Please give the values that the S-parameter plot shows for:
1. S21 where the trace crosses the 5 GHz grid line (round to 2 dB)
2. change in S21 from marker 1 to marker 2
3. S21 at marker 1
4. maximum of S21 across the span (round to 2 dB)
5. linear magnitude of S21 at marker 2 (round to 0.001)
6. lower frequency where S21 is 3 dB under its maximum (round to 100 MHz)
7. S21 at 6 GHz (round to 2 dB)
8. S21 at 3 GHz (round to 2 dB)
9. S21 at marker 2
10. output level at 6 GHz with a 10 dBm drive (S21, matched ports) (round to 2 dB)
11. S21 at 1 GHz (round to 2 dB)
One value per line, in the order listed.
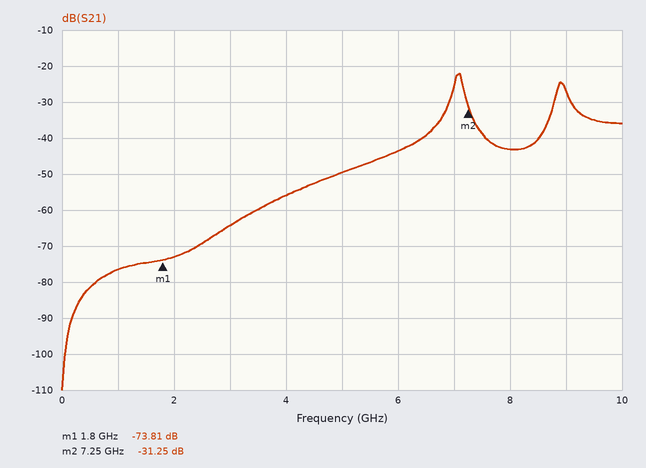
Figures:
-50 dB
42.56 dB
-73.81 dB
-22 dB
0.027
7.0 GHz
-44 dB
-64 dB
-31.25 dB
-34 dBm
-76 dB
